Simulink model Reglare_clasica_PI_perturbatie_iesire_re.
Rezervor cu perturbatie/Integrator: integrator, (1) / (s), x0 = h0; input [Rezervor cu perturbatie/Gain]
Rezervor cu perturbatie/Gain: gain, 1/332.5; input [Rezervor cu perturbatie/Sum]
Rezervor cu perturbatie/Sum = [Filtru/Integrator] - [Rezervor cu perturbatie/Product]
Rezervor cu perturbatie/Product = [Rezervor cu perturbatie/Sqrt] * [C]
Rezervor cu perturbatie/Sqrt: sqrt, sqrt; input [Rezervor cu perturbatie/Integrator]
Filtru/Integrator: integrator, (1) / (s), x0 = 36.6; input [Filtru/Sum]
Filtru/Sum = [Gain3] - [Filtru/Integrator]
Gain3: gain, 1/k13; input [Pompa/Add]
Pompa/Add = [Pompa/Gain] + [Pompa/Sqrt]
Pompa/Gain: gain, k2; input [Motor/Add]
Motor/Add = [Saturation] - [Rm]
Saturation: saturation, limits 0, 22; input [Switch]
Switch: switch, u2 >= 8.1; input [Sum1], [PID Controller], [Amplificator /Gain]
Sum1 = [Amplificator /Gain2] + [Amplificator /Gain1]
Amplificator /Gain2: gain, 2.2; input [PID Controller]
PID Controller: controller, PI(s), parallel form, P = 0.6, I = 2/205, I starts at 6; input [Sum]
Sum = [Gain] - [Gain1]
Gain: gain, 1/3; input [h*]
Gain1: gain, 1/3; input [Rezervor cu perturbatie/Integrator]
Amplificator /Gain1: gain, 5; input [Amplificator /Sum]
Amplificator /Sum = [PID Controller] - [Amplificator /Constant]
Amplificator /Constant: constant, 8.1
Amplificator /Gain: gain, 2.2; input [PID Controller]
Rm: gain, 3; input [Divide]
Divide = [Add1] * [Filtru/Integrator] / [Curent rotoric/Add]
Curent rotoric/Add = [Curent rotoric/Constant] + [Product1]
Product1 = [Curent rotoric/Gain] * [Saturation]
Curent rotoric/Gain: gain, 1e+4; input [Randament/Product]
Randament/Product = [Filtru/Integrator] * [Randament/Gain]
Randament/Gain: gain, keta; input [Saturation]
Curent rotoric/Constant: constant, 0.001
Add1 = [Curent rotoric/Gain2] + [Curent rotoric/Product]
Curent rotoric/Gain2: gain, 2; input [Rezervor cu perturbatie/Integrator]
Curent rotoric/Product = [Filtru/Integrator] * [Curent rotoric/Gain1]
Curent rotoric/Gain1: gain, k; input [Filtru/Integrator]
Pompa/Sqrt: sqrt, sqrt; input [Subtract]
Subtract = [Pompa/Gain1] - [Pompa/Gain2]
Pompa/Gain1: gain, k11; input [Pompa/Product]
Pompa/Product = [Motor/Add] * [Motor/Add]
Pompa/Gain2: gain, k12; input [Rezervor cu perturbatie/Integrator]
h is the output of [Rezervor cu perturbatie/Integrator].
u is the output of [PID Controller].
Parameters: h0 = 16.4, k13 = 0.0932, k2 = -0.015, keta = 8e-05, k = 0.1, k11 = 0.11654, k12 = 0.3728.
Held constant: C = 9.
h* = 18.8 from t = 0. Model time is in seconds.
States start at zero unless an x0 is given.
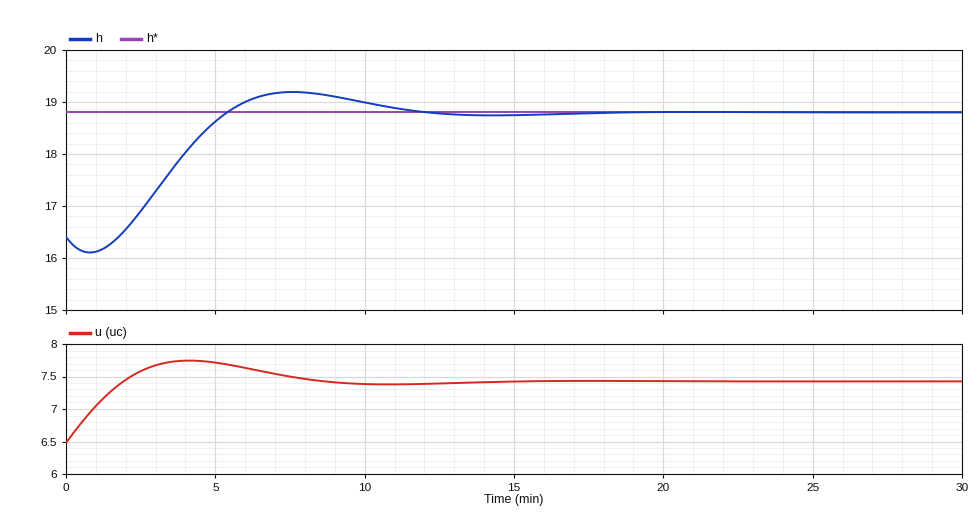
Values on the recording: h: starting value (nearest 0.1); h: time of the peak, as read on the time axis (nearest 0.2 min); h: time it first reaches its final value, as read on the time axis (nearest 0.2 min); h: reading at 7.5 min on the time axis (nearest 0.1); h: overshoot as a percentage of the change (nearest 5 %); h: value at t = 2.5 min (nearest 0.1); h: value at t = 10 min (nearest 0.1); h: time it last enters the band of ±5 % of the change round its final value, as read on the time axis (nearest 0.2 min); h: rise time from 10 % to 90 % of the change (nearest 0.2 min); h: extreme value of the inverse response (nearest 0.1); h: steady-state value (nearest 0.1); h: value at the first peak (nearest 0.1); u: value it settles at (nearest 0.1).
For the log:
16.4
7.6 min
5.4 min
19.2
15 %
16.9
19.0
10.6 min
2.8 min
16.1
18.8
19.2
7.4
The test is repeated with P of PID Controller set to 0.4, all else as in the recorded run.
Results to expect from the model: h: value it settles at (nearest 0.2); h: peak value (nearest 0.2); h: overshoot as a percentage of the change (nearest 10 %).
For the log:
18.8
19.4
30 %
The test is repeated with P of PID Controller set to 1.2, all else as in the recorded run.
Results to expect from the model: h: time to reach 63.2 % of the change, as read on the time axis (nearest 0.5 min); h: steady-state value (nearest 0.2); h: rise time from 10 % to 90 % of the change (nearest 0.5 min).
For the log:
3.5 min
18.8
4.5 min
